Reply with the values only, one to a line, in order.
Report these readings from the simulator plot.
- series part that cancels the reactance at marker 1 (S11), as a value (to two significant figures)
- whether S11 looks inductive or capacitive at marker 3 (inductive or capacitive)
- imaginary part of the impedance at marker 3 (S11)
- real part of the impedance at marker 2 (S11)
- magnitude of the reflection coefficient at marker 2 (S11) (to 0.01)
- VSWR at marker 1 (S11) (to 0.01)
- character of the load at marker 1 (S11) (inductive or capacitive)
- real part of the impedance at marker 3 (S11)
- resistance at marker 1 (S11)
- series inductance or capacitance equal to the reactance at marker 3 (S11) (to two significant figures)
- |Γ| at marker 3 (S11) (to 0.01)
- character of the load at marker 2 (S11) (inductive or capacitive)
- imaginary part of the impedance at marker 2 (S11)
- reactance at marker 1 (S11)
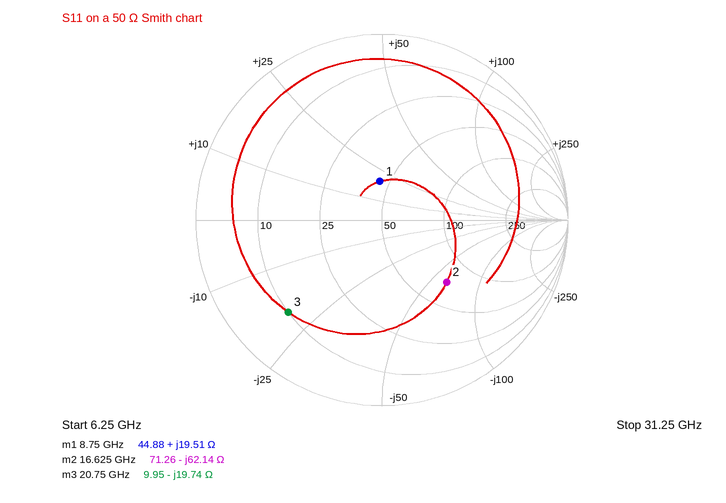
930 fF
capacitive
-19.74 Ω
71.26 Ω
0.48
1.53
inductive
9.95 Ω
44.88 Ω
390 fF
0.71
capacitive
-62.14 Ω
+19.51 Ω
